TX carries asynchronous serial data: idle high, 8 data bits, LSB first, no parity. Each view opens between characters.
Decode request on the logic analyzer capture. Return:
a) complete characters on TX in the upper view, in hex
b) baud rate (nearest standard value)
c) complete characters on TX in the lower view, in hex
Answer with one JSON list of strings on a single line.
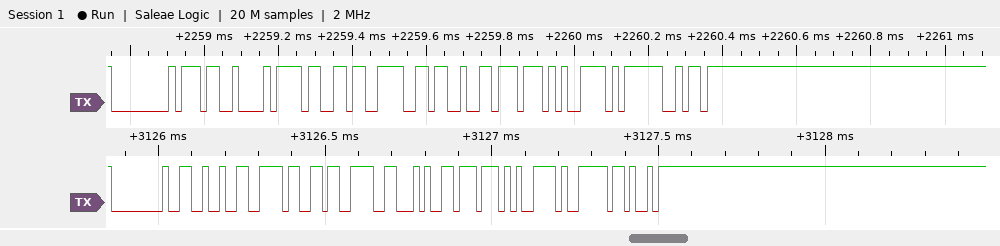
["00, 37, E8, B3, 9E, 93, 77, 79, 3F, FB", "57600 baud", "00, 26, E6, B3, 9E, 94, 77, 79, BE, E9"]
